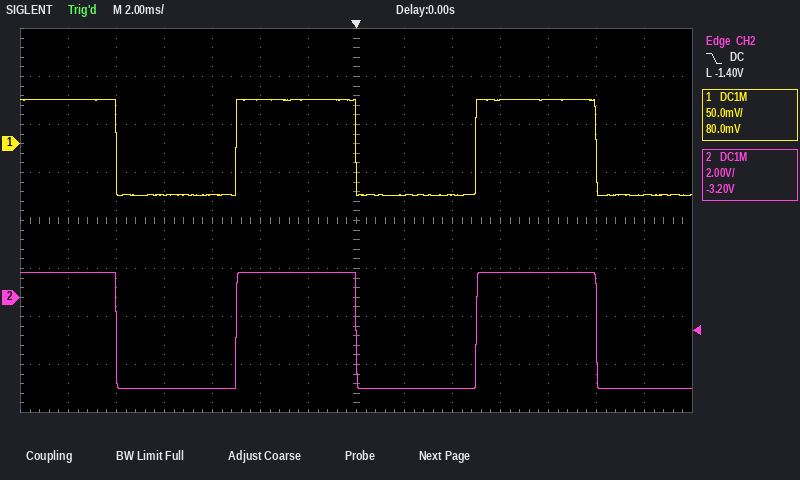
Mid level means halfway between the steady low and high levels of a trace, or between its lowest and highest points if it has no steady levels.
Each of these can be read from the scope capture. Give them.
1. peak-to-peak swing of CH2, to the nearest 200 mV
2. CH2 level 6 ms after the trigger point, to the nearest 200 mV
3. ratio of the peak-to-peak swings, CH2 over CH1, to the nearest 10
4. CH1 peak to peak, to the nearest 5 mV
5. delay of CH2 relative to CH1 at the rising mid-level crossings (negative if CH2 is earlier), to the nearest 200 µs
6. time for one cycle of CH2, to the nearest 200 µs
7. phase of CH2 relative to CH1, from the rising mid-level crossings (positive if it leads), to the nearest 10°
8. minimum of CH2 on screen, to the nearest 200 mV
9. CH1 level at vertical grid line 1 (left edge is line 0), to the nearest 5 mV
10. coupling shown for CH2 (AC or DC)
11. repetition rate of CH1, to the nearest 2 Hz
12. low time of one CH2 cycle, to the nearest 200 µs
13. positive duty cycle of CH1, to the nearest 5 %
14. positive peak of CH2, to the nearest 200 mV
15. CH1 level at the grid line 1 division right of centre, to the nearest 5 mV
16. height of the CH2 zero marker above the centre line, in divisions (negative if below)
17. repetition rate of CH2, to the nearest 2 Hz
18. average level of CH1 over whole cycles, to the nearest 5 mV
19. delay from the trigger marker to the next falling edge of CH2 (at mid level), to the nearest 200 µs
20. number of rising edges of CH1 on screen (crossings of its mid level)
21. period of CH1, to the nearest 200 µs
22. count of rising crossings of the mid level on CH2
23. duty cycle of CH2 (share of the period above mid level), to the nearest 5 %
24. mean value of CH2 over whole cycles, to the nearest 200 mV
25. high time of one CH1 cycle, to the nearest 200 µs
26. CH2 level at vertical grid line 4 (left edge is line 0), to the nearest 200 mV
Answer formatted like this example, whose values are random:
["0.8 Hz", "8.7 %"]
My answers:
["4.8 V", "1.0 V", "50", "100 mV", "0.0 ms", "10.0 ms", "0°", "-3.8 V", "45 mV", "DC", "100 Hz", "5.0 ms", "50 %", "1.0 V", "-55 mV", "-1.6 div", "100 Hz", "-5 mV", "10.0 ms", "2", "10.0 ms", "2", "50 %", "-1.4 V", "5.0 ms", "-3.8 V"]
